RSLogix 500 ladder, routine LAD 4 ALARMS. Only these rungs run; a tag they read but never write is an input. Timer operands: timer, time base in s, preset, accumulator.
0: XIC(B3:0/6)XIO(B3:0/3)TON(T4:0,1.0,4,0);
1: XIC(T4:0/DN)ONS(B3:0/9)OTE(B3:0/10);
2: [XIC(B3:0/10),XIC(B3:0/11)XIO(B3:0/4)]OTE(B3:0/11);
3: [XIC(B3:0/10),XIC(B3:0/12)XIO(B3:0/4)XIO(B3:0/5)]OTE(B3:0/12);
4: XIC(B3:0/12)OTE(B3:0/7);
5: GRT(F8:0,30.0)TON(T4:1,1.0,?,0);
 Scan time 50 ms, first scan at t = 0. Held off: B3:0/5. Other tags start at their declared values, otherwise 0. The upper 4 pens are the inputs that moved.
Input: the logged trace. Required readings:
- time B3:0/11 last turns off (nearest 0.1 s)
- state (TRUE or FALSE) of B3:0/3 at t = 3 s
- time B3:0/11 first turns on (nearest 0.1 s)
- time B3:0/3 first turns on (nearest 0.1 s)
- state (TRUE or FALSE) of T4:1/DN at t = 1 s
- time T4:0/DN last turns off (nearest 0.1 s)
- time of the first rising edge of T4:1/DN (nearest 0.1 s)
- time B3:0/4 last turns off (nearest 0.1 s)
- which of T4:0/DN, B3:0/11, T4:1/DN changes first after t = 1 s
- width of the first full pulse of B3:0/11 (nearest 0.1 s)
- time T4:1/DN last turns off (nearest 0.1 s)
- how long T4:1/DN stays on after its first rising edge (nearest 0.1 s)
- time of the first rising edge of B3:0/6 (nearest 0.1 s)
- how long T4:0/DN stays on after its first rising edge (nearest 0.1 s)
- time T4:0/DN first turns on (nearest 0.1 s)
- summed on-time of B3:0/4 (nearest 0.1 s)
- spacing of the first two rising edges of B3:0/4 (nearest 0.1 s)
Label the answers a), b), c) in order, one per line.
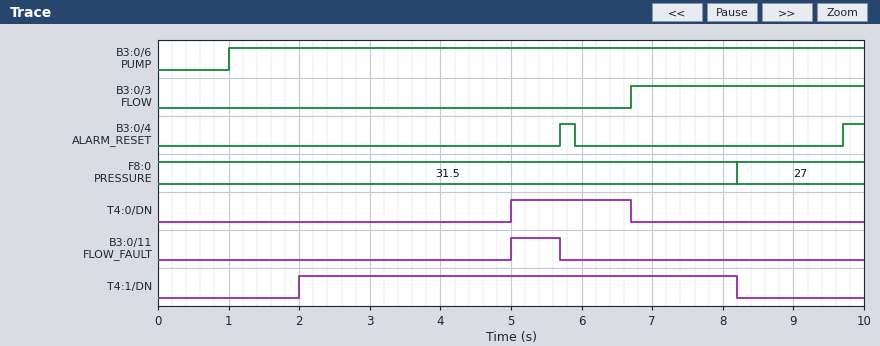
a) 5.7 s
b) FALSE
c) 5.0 s
d) 6.7 s
e) FALSE
f) 6.7 s
g) 2.0 s
h) 5.9 s
i) T4:1/DN
j) 0.7 s
k) 8.2 s
l) 6.2 s
m) 1.0 s
n) 1.7 s
o) 5.0 s
p) 0.5 s
q) 4.0 s
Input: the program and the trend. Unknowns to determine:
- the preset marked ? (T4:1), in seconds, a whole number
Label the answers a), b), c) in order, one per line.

a) 2 s
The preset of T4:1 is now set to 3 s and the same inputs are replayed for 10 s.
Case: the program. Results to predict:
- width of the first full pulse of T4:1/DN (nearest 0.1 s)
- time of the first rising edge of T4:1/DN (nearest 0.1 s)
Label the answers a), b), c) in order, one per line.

a) 5.2 s
b) 3.0 s
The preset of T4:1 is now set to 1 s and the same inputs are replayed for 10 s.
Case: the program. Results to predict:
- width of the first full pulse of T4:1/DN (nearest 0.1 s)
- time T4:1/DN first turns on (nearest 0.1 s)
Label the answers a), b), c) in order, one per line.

a) 7.2 s
b) 1.0 s
